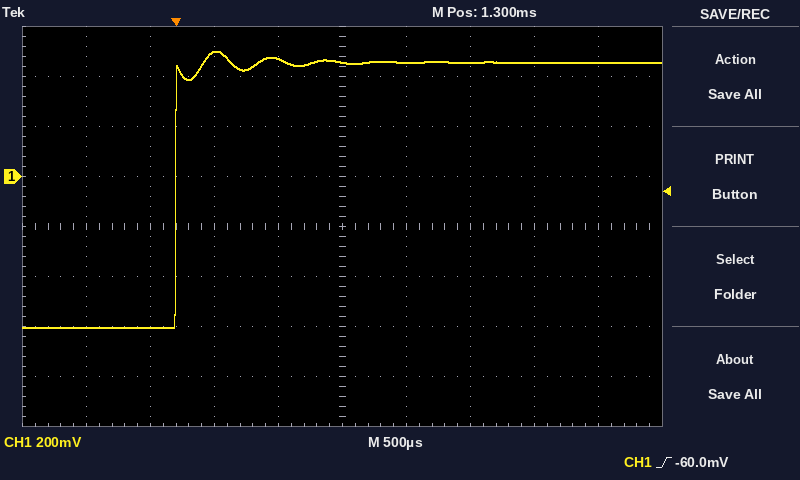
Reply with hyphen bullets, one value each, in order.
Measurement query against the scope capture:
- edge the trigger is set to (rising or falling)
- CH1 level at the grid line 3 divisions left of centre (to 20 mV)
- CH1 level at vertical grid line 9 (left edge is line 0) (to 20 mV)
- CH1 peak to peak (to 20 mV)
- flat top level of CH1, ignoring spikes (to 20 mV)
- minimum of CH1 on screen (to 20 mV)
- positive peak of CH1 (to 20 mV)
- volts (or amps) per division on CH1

- rising
- -600 mV
- 460 mV
- 1.10 V
- 460 mV
- -600 mV
- 500 mV
- 200 mV
